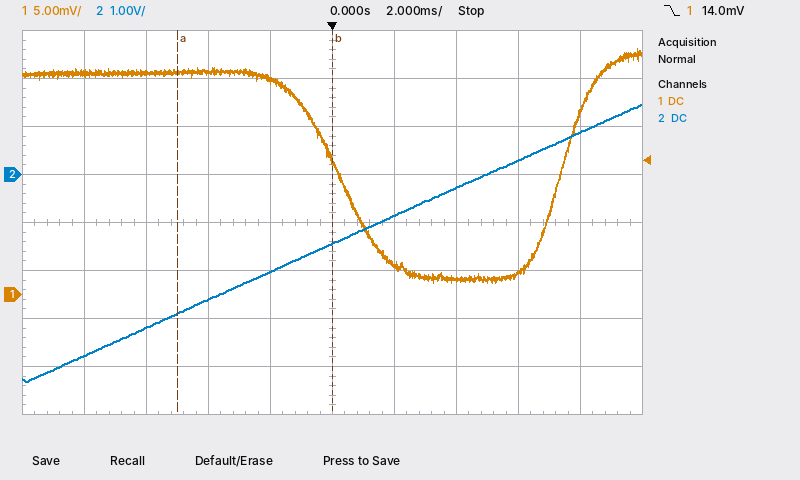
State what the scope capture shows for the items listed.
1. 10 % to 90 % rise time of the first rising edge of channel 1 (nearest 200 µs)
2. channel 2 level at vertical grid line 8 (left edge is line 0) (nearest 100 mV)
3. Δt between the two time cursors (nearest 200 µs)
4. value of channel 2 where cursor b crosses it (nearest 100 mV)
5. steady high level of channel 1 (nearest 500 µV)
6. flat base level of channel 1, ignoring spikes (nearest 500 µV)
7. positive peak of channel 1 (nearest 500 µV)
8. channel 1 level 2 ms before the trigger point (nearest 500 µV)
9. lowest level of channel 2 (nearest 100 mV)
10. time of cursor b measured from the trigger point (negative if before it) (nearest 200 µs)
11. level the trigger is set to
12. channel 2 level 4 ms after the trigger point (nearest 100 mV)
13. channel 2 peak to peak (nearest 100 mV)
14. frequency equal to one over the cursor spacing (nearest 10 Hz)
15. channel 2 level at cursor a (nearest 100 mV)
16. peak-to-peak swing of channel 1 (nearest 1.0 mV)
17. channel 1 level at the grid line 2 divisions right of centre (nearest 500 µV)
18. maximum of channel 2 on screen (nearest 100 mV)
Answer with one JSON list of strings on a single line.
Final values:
["1.8 ms", "300 mV", "5.0 ms", "-1.4 V", "23.0 mV", "1.5 mV", "25.5 mV", "22.5 mV", "-4.3 V", "0.0 ms", "14.0 mV", "-300 mV", "5.8 V", "200 Hz", "-2.9 V", "24.0 mV", "1.5 mV", "1.5 V"]
